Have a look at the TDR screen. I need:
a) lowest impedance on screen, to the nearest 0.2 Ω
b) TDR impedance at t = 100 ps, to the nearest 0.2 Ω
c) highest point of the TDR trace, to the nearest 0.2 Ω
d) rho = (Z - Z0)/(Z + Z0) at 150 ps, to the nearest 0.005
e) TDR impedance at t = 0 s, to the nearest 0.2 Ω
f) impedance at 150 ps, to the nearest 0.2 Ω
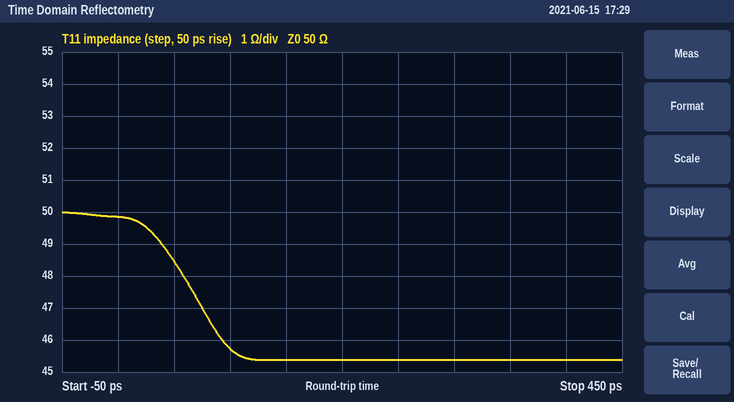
45.4 Ω
45.8 Ω
50.0 Ω
-0.050
49.8 Ω
45.4 Ω
